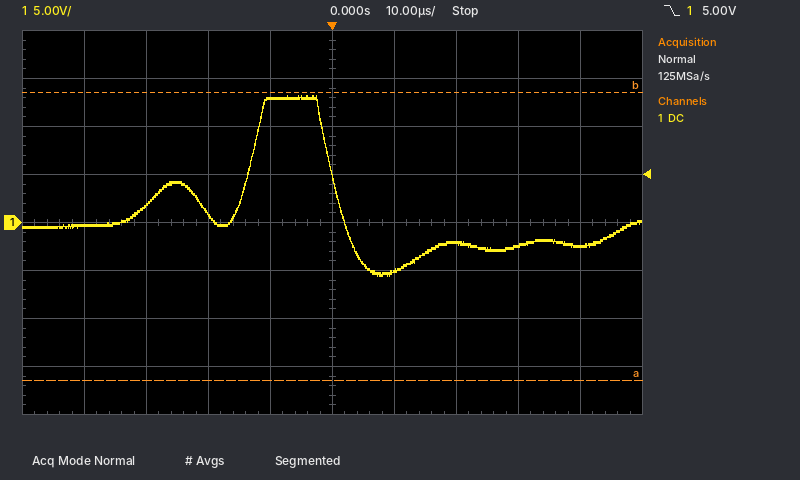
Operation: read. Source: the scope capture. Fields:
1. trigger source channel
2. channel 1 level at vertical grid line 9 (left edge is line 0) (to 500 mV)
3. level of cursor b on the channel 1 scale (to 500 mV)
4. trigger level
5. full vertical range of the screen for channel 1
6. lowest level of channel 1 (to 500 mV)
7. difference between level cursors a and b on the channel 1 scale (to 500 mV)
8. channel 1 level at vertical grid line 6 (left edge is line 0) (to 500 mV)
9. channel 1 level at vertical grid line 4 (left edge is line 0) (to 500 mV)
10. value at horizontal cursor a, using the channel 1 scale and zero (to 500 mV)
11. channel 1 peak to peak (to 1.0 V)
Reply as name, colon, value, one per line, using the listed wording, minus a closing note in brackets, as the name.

trigger source channel: channel 1
channel 1 level at vertical grid line 9 (left edge is line 0): -2.5 V
level of cursor b on the channel 1 scale: 13.5 V
trigger level: 5.00 V
full vertical range of the screen for channel 1: 40 V
lowest level of channel 1: -5.5 V
difference between level cursors a and b on the channel 1 scale: 30.0 V
channel 1 level at vertical grid line 6 (left edge is line 0): -5.0 V
channel 1 level at vertical grid line 4 (left edge is line 0): 13.0 V
value at horizontal cursor a, using the channel 1 scale and zero: -16.5 V
channel 1 peak to peak: 19.0 V
